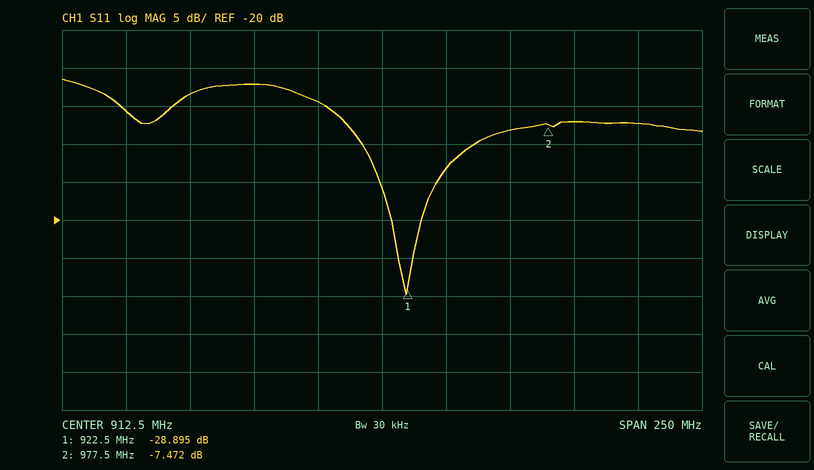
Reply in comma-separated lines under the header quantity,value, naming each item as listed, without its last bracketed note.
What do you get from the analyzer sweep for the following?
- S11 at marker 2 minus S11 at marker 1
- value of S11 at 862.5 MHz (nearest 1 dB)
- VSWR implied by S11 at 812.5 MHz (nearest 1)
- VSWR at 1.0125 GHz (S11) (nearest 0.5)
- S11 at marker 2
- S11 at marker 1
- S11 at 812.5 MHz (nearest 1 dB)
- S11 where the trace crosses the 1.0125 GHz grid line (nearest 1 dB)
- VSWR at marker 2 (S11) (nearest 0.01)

quantity,value
S11 at marker 2 minus S11 at marker 1,21.423 dB
value of S11 at 862.5 MHz,-2 dB
VSWR implied by S11 at 812.5 MHz,3
VSWR at 1.0125 GHz (S11),2.5
S11 at marker 2,-7.472 dB
S11 at marker 1,-28.895 dB
S11 at 812.5 MHz,-6 dB
S11 where the trace crosses the 1.0125 GHz grid line,-7 dB
VSWR at marker 2 (S11),2.47
